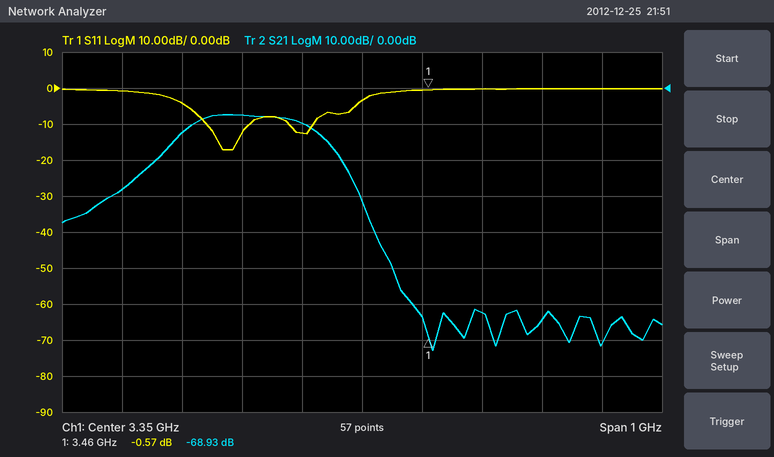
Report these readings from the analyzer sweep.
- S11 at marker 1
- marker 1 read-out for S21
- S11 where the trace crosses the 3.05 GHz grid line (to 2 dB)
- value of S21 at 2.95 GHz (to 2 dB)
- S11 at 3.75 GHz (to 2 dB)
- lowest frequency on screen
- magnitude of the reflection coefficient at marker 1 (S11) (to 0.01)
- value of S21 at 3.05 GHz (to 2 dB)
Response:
-0.57 dB
-68.93 dB
-4 dB
-28 dB
0 dB
2.85 GHz
0.94
-12 dB
